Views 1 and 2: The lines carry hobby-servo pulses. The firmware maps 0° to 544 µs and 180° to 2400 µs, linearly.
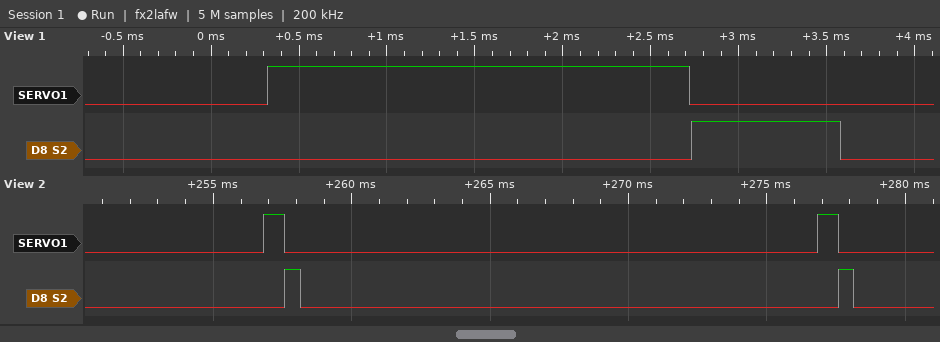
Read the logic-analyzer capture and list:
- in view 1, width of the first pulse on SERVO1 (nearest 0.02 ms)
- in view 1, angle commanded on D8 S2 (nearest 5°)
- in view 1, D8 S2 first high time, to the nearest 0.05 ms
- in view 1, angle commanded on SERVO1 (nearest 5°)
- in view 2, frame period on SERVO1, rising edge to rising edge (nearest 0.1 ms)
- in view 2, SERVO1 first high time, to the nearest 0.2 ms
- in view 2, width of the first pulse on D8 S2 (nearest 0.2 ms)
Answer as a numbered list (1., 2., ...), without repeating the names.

1. 2.40 ms
2. 30°
3. 0.85 ms
4. 180°
5. 20.0 ms
6. 0.8 ms
7. 0.6 ms
